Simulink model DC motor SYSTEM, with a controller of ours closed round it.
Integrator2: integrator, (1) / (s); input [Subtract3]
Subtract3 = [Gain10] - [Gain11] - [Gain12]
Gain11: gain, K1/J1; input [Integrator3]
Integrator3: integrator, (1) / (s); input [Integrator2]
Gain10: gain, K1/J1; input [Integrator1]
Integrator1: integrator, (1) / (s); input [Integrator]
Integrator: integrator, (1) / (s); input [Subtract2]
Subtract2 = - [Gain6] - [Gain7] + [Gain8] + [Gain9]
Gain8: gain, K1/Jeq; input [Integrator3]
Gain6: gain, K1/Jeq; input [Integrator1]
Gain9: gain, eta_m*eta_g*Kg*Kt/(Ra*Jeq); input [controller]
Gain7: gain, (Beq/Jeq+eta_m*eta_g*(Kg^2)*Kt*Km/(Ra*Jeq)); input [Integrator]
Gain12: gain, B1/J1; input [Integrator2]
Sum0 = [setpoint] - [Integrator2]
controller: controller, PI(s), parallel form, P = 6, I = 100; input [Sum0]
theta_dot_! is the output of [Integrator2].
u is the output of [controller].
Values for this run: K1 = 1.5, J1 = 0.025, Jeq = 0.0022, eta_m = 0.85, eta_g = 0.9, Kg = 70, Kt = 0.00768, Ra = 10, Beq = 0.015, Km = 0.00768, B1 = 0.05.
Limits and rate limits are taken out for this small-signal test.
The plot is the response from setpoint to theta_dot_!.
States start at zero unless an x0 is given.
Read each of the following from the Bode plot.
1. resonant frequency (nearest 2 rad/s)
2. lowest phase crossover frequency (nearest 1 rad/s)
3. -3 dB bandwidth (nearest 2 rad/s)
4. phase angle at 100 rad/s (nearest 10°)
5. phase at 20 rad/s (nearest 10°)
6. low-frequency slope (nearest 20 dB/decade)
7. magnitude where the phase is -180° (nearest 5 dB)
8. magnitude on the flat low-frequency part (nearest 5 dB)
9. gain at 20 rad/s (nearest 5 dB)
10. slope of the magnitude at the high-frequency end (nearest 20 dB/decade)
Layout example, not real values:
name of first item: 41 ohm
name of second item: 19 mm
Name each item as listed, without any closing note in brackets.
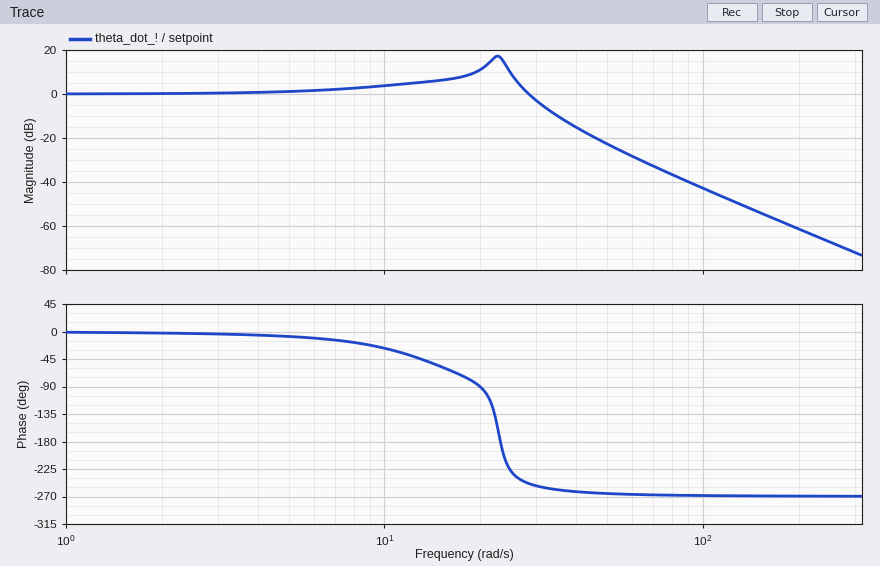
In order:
resonant frequency: 22 rad/s
lowest phase crossover frequency: 23 rad/s
-3 dB bandwidth: 30 rad/s
phase angle at 100 rad/s: -270°
phase at 20 rad/s: -90°
low-frequency slope: 0 dB/decade
magnitude where the phase is -180°: 15 dB
magnitude on the flat low-frequency part: 0 dB
gain at 20 rad/s: 10 dB
slope of the magnitude at the high-frequency end: -60 dB/decade
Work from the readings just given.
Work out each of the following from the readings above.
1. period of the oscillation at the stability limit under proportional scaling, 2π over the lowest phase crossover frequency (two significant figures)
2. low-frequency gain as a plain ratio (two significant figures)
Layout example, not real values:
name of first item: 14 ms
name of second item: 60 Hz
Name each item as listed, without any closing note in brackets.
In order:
period of the oscillation at the stability limit under proportional scaling, 2π over the lowest phase crossover frequency: 0.27 s
low-frequency gain as a plain ratio: 1.0
